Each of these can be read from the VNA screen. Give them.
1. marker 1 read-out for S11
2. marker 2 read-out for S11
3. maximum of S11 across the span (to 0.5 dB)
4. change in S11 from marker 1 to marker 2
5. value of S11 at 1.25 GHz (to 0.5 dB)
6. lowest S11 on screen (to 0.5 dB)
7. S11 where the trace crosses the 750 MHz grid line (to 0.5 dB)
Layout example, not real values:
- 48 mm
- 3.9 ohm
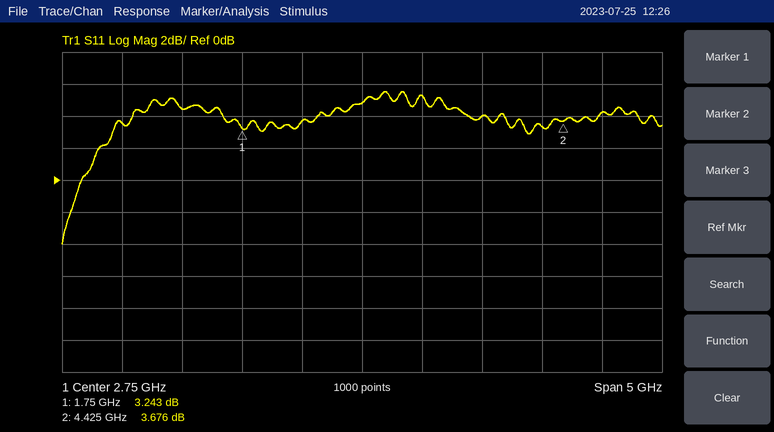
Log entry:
- 3.243 dB
- 3.676 dB
- 5.5 dB
- 0.433 dB
- 4.5 dB
- -4.0 dB
- 3.5 dB
